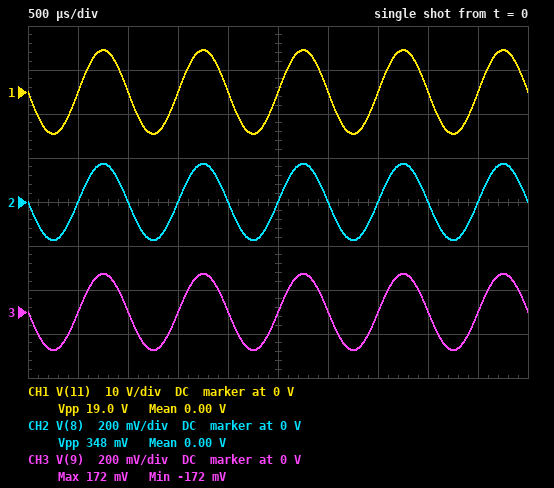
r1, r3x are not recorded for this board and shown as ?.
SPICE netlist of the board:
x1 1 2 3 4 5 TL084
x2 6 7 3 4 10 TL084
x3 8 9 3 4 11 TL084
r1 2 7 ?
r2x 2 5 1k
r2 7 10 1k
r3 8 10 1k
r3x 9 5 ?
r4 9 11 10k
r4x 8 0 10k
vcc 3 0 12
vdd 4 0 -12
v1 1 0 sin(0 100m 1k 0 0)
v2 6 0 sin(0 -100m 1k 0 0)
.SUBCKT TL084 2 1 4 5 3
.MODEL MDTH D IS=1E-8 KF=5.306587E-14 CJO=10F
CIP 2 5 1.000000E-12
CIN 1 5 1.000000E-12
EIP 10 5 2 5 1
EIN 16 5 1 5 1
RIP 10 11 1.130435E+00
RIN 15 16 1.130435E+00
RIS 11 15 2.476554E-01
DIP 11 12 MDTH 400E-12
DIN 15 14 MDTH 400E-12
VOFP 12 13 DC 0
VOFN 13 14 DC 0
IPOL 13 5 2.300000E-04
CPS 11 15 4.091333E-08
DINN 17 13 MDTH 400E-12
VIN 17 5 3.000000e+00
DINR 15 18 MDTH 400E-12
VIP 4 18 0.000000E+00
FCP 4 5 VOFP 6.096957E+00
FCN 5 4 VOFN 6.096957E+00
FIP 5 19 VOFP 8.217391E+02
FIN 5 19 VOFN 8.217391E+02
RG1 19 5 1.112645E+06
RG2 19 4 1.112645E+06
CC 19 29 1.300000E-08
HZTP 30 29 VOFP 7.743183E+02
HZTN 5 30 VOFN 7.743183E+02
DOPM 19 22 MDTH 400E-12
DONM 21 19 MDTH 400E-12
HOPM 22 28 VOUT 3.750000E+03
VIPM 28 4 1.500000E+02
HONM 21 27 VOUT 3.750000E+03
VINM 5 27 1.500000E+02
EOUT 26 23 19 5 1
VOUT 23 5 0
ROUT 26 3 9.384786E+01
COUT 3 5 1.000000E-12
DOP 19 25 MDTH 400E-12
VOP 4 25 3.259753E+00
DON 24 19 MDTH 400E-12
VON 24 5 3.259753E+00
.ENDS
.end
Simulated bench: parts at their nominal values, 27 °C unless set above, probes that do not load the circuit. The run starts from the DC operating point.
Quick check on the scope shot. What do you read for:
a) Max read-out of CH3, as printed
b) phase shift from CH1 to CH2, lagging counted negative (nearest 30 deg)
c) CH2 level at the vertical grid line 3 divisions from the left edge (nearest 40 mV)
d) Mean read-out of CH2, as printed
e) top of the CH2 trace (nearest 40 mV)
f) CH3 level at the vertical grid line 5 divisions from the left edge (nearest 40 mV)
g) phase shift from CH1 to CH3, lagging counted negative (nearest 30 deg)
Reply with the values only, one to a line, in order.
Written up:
172 mV
0 deg
0 V
0.00 V
160 mV
0 V
0 deg
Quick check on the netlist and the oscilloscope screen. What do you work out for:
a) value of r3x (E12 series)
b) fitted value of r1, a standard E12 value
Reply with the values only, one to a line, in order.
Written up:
390 Ω
2.2 kΩ
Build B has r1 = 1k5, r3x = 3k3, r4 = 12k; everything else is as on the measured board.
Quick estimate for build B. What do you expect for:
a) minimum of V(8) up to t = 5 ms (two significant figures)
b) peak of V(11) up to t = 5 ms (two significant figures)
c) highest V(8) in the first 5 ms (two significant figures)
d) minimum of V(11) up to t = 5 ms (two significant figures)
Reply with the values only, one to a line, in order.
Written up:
-210 mV
1.8 V
210 mV
-1.8 V
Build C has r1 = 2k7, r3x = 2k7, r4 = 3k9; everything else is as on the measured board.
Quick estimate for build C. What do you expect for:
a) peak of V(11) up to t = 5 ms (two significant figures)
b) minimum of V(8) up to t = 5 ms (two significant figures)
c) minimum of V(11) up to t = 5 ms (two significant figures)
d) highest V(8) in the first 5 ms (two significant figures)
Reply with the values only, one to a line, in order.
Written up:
640 mV
-160 mV
-640 mV
160 mV
